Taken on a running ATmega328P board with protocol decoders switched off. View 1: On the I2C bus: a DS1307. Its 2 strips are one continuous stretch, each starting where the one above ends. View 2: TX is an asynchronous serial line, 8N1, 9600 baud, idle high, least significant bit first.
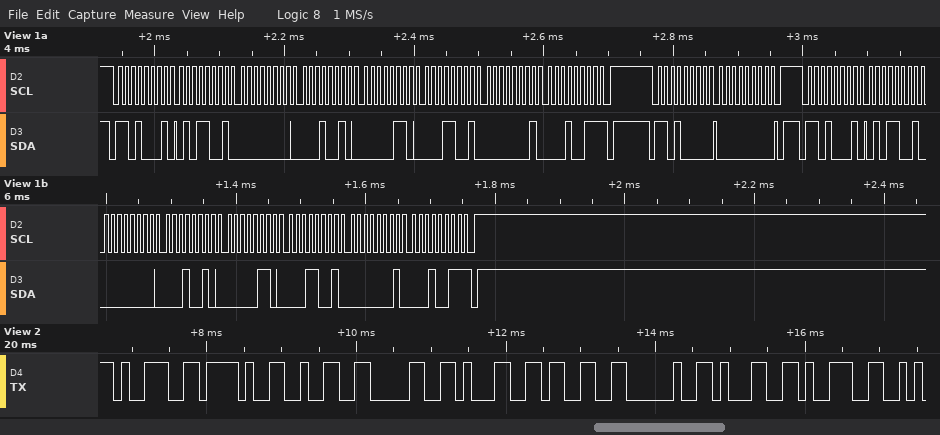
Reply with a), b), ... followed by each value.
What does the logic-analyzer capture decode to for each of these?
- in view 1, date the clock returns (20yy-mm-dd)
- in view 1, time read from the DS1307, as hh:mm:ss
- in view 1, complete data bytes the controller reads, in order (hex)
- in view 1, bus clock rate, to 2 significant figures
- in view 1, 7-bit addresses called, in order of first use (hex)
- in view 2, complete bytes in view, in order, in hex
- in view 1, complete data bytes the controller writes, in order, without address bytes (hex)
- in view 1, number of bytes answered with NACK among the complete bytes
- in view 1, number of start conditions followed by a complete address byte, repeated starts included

a) 2013-01-19
b) 12:00:59
c) 59 00 12 06 19 01 13 59 00 12 06 19 01 13
d) 100 kHz
e) 0x68
f) 39 2F 32 30 31 33 20 31 39
g) 00
h) 2
i) 3
